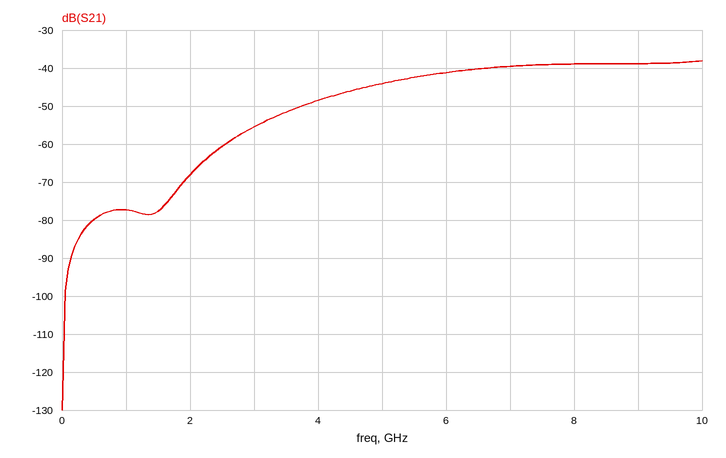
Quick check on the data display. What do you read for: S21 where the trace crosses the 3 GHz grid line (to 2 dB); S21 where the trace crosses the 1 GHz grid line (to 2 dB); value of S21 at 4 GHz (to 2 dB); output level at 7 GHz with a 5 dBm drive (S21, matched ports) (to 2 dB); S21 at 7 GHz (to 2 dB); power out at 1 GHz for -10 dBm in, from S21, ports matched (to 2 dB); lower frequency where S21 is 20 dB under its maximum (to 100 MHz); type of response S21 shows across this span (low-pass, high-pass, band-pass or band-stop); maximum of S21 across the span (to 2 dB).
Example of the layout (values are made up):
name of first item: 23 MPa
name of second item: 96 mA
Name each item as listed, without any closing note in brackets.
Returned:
S21 where the trace crosses the 3 GHz grid line: -56 dB
S21 where the trace crosses the 1 GHz grid line: -78 dB
value of S21 at 4 GHz: -48 dB
output level at 7 GHz with a 5 dBm drive (S21, matched ports): -34 dBm
S21 at 7 GHz: -40 dB
power out at 1 GHz for -10 dBm in, from S21, ports matched: -88 dBm
lower frequency where S21 is 20 dB under its maximum: 2.7 GHz
type of response S21 shows across this span: high-pass
maximum of S21 across the span: -38 dB
